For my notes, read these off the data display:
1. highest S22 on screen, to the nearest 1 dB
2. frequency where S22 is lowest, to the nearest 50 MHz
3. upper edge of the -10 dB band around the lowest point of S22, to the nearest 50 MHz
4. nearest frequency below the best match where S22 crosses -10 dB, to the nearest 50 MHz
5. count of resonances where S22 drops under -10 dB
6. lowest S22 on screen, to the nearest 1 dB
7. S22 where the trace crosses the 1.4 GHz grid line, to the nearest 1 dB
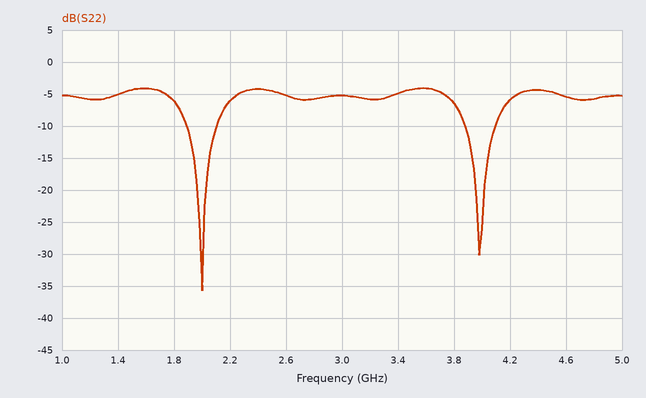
-4 dB
2.00 GHz
2.10 GHz
1.90 GHz
2
-36 dB
-5 dB
